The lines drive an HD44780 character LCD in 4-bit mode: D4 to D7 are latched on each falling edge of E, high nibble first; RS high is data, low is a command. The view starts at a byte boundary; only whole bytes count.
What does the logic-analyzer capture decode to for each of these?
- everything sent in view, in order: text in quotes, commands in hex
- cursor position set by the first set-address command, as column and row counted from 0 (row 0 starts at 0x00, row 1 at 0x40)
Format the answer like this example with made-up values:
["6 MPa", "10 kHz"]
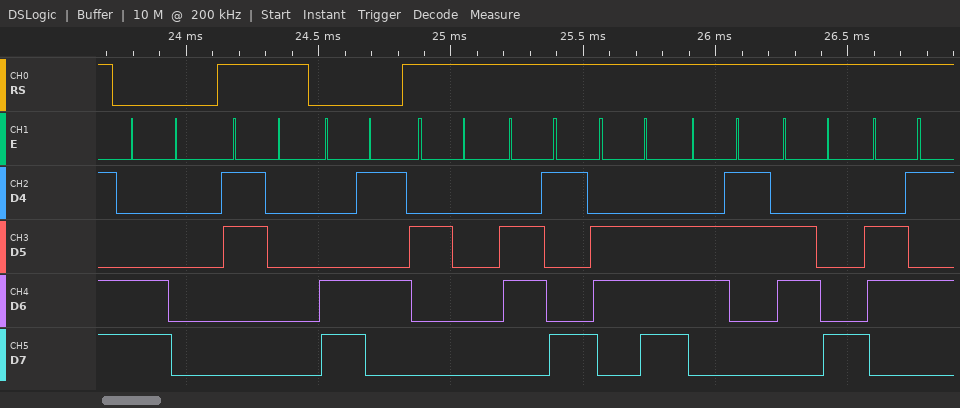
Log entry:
["0xC0 \"0\" 0xC5 \" inche\"", "column 0, row 1"]
